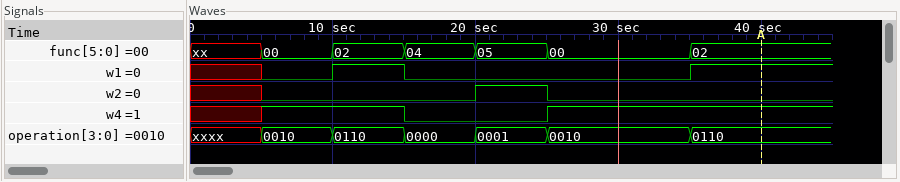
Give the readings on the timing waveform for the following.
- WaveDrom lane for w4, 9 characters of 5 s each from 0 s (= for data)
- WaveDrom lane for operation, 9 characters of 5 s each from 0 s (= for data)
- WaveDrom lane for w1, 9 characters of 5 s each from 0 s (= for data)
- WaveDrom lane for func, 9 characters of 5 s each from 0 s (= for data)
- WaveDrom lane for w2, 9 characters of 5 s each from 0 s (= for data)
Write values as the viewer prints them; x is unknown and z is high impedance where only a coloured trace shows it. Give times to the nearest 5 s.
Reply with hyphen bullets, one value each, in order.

- {name: 'w4', wave: 'x1.0.1...'}
- {name: 'operation', wave: 'x=====.=.', data: '0010 0110 0000 0001 0010 0110'}
- {name: 'w1', wave: 'x010...1.'}
- {name: 'func', wave: 'x=====.=.', data: '00 02 04 05 00 02'}
- {name: 'w2', wave: 'x0..10...'}
